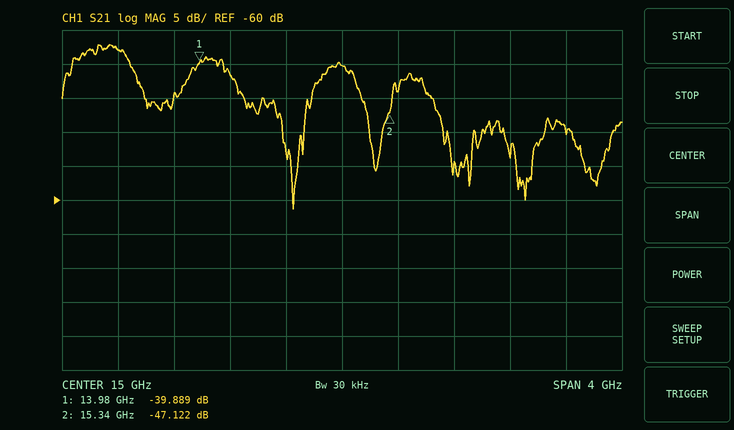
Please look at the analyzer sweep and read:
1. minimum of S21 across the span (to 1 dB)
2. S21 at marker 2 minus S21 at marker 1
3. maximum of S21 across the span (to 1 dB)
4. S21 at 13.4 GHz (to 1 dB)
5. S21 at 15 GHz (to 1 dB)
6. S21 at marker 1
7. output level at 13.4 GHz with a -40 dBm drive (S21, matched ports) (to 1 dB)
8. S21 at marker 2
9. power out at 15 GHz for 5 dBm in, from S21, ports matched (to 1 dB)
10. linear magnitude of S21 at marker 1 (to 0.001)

-61 dB
-7.233 dB
-37 dB
-38 dB
-40 dB
-39.889 dB
-78 dBm
-47.122 dB
-35 dBm
0.010
